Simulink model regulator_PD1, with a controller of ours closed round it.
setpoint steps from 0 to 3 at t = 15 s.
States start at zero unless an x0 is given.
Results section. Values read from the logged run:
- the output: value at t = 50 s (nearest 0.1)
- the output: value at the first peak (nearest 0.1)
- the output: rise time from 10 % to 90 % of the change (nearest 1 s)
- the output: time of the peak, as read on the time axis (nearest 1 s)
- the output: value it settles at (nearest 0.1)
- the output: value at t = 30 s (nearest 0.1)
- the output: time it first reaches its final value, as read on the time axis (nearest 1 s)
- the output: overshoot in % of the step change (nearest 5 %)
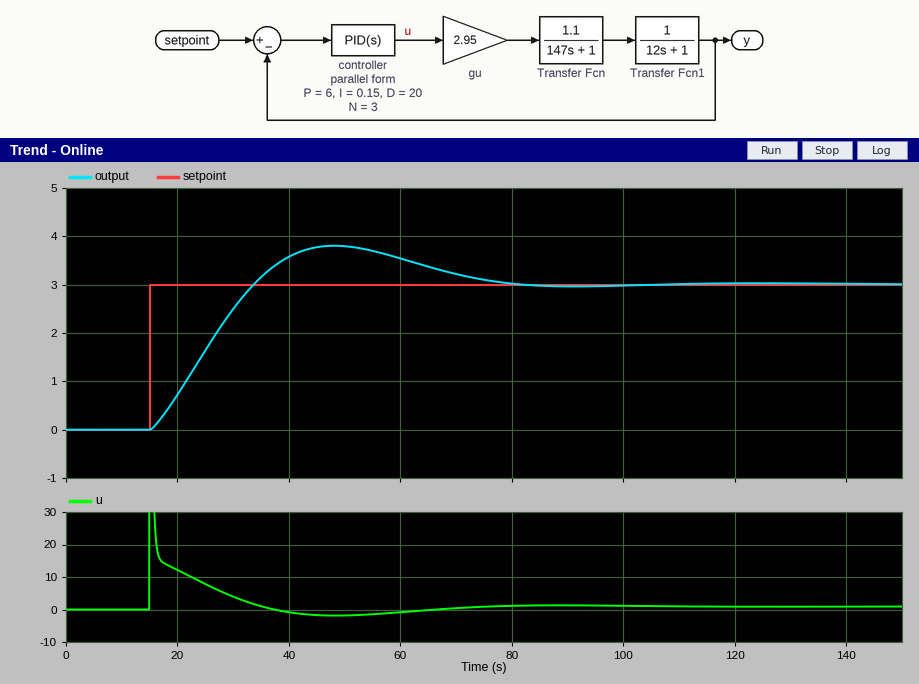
3.8
3.8
14 s
48 s
3.0
2.5
34 s
25 %
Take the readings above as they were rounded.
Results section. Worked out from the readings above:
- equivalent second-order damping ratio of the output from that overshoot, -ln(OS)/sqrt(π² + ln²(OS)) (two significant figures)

0.40
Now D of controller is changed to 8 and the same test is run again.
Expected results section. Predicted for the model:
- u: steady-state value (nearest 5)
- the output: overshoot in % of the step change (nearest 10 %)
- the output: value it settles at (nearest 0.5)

0
40 %
3.0
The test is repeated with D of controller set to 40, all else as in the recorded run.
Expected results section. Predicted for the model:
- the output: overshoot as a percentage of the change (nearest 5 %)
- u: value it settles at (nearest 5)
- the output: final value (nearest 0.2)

15 %
0
3.0
